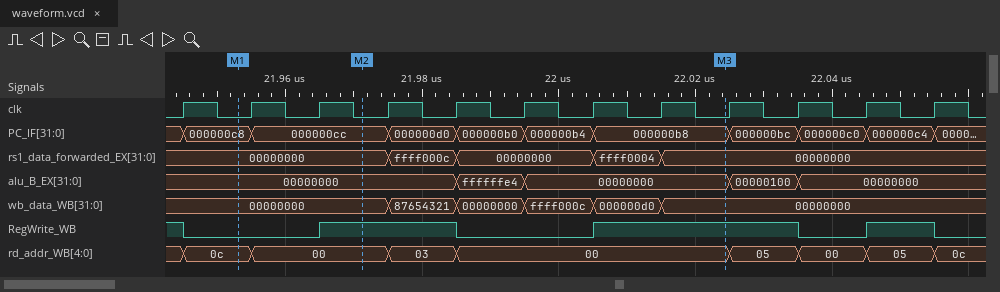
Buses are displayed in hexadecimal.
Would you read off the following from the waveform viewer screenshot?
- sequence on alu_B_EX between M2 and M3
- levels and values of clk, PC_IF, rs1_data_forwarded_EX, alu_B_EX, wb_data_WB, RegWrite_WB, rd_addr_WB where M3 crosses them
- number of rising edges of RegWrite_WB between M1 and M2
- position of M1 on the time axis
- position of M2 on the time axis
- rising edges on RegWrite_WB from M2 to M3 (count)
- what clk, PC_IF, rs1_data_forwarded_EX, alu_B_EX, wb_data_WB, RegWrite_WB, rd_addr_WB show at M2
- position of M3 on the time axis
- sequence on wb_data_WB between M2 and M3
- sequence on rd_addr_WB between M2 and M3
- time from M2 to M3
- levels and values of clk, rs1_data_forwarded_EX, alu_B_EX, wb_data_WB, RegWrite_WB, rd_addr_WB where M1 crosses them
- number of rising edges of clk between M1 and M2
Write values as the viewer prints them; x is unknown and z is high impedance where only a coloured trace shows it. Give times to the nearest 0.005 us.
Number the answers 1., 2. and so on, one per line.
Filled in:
1. 00000000, ffffffe4, 00000000
2. clk=0, PC_IF=000000b8, rs1_data_forwarded_EX=00000000, alu_B_EX=00000000, wb_data_WB=00000000, RegWrite_WB=1, rd_addr_WB=00
3. 1
4. 21.955 us
5. 21.97 us
6. 1
7. clk=0, PC_IF=000000cc, rs1_data_forwarded_EX=00000000, alu_B_EX=00000000, wb_data_WB=00000000, RegWrite_WB=1, rd_addr_WB=00
8. 22.025 us
9. 00000000, 87654321, 00000000, ffff000c, 000000d0, 00000000
10. 00, 03, 00
11. 0.055 us
12. clk=0, rs1_data_forwarded_EX=00000000, alu_B_EX=00000000, wb_data_WB=00000000, RegWrite_WB=0, rd_addr_WB=0c
13. 2
